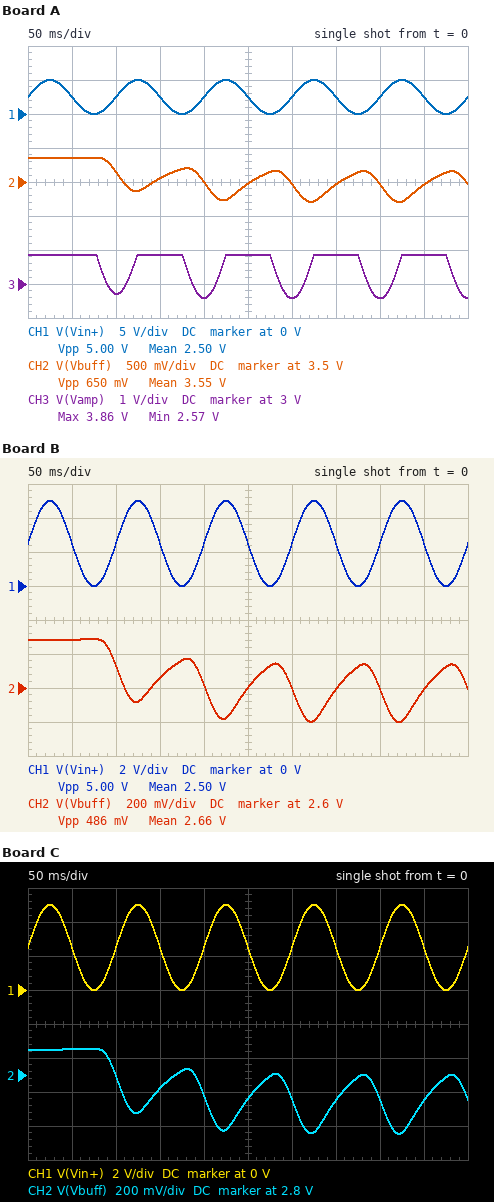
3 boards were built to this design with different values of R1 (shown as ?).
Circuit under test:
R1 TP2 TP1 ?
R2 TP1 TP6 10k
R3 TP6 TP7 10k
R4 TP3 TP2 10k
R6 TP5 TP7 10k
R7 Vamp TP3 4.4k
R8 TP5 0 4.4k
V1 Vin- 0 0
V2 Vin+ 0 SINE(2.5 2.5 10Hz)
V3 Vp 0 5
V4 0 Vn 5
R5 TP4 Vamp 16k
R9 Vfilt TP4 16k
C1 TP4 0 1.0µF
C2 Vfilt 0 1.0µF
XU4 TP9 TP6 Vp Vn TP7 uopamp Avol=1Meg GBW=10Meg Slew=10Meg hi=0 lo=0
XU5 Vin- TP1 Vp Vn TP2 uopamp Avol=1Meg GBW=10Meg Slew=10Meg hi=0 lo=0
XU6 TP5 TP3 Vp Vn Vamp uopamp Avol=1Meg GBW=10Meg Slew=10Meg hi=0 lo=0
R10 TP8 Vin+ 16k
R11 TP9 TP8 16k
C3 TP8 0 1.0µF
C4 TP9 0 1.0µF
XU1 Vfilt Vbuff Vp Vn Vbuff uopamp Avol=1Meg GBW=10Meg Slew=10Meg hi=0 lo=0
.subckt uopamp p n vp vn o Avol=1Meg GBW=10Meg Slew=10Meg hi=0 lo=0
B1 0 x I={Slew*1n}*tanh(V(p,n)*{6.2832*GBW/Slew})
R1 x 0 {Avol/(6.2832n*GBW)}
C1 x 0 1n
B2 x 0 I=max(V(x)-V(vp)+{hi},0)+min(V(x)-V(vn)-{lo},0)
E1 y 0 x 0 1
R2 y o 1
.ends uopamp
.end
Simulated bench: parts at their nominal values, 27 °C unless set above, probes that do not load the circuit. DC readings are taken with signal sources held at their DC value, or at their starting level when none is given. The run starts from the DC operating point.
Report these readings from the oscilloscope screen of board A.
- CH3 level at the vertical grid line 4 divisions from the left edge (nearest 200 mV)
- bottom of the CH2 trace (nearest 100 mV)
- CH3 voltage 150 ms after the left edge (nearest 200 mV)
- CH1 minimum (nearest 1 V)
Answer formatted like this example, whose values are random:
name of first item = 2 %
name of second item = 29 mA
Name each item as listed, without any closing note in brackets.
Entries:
CH3 level at the vertical grid line 4 divisions from the left edge = 2.6 V
bottom of the CH2 trace = 3.2 V
CH3 voltage 150 ms after the left edge = 3.8 V
CH1 minimum = 0 V
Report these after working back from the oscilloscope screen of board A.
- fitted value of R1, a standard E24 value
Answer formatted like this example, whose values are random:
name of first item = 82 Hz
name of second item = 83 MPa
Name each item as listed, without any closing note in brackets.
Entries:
fitted value of R1, a standard E24 value = 15 kΩ
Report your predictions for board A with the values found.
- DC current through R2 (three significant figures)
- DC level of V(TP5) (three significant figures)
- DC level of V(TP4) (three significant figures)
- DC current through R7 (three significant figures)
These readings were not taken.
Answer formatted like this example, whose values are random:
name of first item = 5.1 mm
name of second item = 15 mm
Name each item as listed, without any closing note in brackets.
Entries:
DC current through R2 = 250 µA
DC level of V(TP5) = 1.53 V
DC level of V(TP4) = 3.85 V
DC current through R7 = 528 µA
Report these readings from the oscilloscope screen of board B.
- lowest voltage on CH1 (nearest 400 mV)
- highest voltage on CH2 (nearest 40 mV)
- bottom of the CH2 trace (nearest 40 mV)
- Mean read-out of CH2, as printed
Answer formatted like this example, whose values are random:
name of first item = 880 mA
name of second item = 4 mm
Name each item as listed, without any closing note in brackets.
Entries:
lowest voltage on CH1 = 0 V
highest voltage on CH2 = 2.88 V
bottom of the CH2 trace = 2.40 V
Mean read-out of CH2, as printed = 2.66 V
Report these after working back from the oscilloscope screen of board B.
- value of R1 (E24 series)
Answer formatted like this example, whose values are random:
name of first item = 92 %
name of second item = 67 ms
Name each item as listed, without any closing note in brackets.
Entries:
value of R1 = 6.2 kΩ
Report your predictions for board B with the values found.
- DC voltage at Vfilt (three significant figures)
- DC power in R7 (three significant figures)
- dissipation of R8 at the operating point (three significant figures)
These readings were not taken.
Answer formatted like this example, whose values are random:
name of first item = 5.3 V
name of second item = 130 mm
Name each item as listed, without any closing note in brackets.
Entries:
DC voltage at Vfilt = 2.88 V
DC power in R7 = 417 µW
dissipation of R8 at the operating point = 530 µW
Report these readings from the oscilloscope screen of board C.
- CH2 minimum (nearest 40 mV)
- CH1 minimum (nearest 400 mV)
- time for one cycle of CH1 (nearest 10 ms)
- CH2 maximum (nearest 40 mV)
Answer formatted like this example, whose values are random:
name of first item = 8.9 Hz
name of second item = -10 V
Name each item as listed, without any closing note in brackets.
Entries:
CH2 minimum = 2.44 V
CH1 minimum = 0 V
time for one cycle of CH1 = 100 ms
CH2 maximum = 2.96 V
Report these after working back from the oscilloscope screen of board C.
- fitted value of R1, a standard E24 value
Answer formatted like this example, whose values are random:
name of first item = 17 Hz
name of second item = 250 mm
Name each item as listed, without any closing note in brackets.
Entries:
fitted value of R1, a standard E24 value = 6.8 kΩ
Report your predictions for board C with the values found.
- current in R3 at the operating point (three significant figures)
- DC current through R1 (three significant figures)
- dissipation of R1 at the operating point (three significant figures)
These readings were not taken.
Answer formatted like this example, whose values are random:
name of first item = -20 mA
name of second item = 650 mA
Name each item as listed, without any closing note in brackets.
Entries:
current in R3 at the operating point = 250 µA
DC current through R1 = 250 µA
dissipation of R1 at the operating point = 425 µW
